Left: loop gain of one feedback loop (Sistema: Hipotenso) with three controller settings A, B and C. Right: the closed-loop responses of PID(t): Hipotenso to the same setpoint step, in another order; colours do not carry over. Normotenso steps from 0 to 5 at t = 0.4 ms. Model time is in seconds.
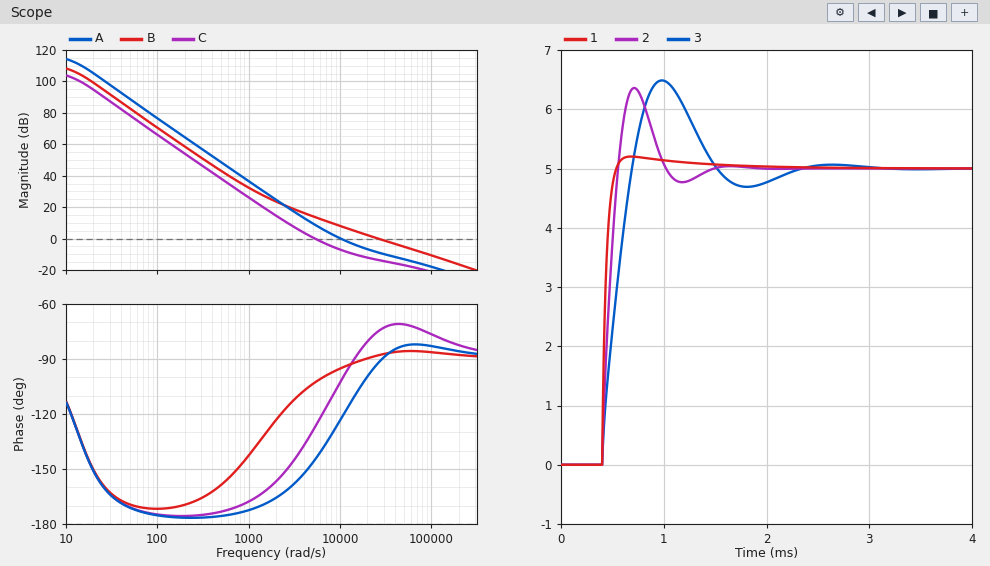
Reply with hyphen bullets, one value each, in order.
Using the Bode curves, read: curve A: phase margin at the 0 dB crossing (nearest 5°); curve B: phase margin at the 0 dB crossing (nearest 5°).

- 55°
- 90°
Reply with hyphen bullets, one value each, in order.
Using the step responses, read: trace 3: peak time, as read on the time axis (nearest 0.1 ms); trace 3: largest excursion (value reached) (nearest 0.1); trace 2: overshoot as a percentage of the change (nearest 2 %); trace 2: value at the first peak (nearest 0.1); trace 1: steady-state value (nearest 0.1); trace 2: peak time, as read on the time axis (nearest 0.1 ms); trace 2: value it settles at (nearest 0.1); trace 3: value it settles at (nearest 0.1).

- 1.0 ms
- 6.5
- 28 %
- 6.4
- 5.0
- 0.7 ms
- 5.0
- 5.0
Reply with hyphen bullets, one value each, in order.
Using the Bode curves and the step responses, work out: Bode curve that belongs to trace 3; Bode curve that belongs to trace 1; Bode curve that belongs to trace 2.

- C
- B
- A
